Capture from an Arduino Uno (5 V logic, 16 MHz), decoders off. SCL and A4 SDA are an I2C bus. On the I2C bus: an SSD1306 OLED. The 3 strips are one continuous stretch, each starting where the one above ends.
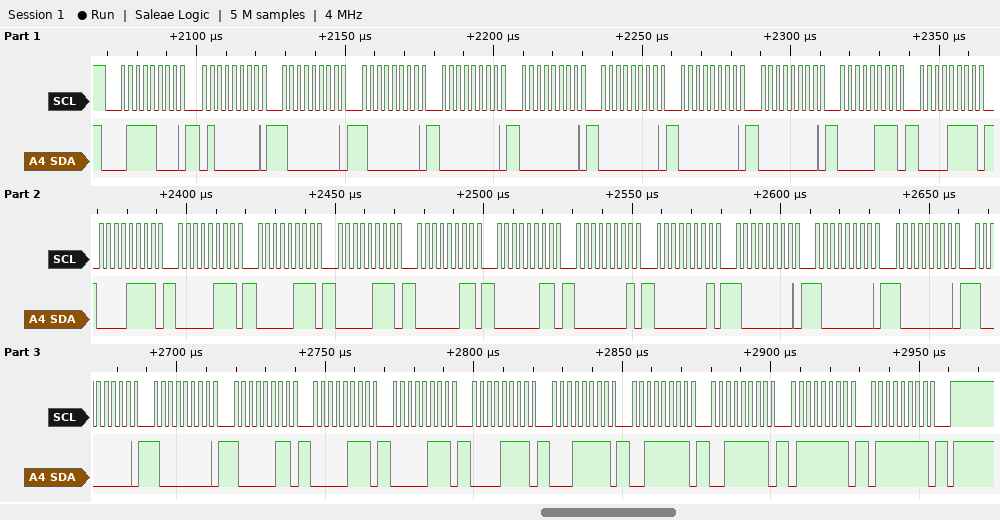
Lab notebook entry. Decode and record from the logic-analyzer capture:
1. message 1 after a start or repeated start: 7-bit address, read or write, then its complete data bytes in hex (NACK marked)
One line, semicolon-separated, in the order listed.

0x3C write: 40 80 80 00 00 00 00 00 07 0F 0F 07 07 07 03 03 01 01 80 80 80 80 80 83 07 07 0F 1F 3F 3F 7F 7F
